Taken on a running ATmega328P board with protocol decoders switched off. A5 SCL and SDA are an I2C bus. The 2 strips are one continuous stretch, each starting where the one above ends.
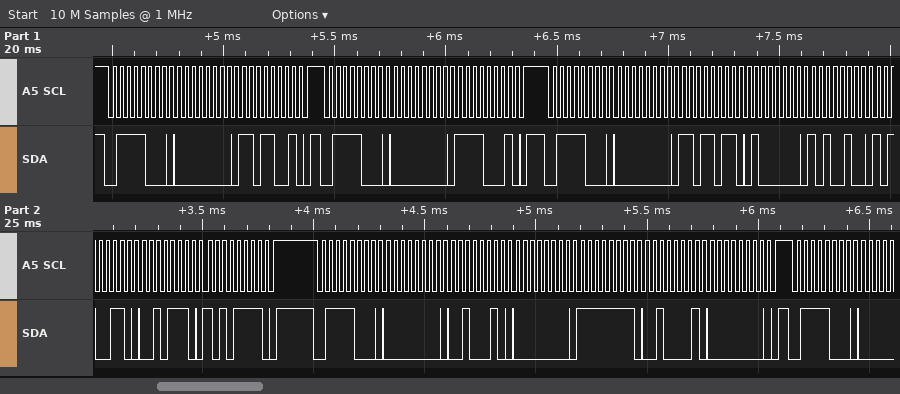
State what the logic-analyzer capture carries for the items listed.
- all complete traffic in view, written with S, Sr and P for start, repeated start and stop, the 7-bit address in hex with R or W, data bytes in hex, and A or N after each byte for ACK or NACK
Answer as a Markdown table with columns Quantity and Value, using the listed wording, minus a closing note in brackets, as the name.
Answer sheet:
| Quantity | Value |
|---|---|
| all complete traffic in view, written with S, Sr and P for start, repeated start and stop, the 7-bit address in hex with R or W, data bytes in hex, and A or N after each byte for ACK or NACK | S 3CW A 00 A D9 A P S 3CW A 00 A F1 A P S 3CW A 00 A DB A 40 A A4 A A6 A 2E A AF A P S 3CW A 00 A 22 A 00 A FF A 21 A 00 A P S 3CW A |
